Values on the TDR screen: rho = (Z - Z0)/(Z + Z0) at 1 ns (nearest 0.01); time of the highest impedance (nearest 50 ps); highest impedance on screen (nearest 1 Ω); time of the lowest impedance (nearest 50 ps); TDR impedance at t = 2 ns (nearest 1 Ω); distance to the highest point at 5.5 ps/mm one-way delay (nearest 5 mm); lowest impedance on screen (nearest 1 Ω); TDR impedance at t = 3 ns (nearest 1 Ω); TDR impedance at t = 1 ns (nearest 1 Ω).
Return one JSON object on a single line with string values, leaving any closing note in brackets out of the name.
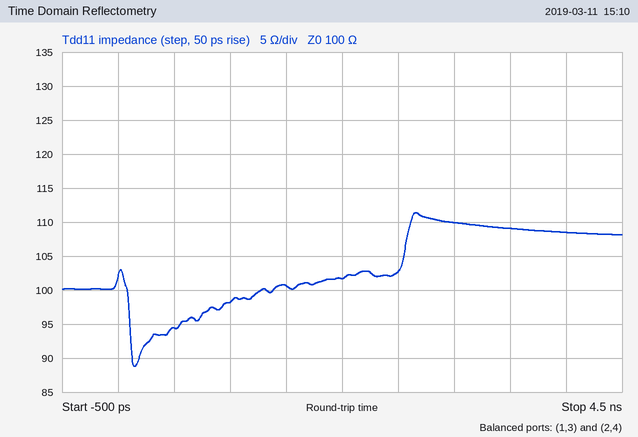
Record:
{"rho = (Z - Z0)/(Z + Z0) at 1 ns": "-0.01", "time of the highest impedance": "2.65 ns", "highest impedance on screen": "111 Ω", "time of the lowest impedance": "150 ps", "TDR impedance at t = 2 ns": "102 Ω", "distance to the highest point at 5.5 ps/mm one-way delay": "240 mm", "lowest impedance on screen": "89 Ω", "TDR impedance at t = 3 ns": "110 Ω", "TDR impedance at t = 1 ns": "98 Ω"}
